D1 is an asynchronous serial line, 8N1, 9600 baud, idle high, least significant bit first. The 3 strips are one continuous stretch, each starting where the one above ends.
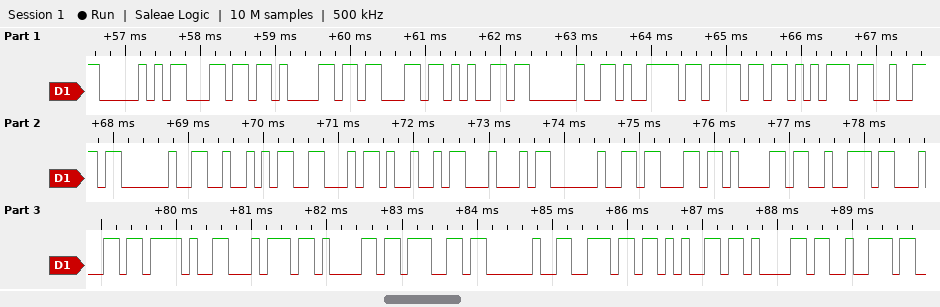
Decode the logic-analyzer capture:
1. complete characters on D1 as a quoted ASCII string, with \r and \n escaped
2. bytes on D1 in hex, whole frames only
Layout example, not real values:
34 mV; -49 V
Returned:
"Place your RFID card/tag near"; 50 6C 61 63 65 20 79 6F 75 72 20 52 46 49 44 20 63 61 72 64 2F 74 61 67 20 6E 65 61 72
